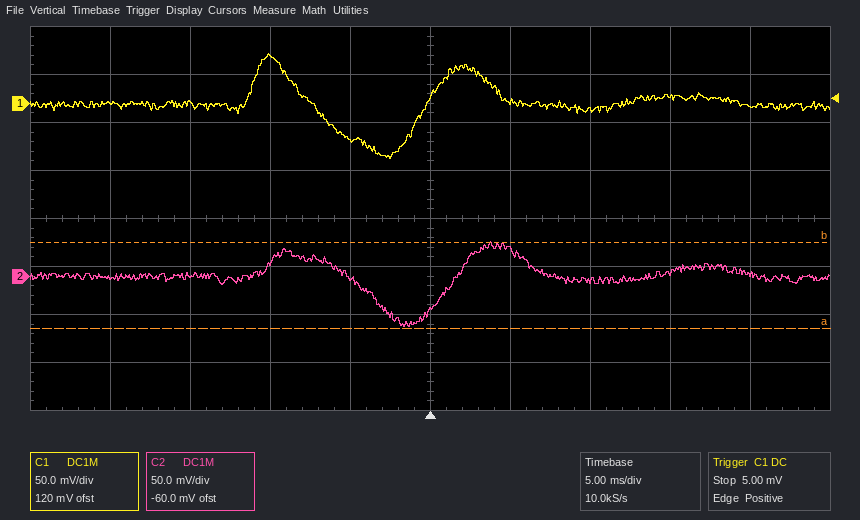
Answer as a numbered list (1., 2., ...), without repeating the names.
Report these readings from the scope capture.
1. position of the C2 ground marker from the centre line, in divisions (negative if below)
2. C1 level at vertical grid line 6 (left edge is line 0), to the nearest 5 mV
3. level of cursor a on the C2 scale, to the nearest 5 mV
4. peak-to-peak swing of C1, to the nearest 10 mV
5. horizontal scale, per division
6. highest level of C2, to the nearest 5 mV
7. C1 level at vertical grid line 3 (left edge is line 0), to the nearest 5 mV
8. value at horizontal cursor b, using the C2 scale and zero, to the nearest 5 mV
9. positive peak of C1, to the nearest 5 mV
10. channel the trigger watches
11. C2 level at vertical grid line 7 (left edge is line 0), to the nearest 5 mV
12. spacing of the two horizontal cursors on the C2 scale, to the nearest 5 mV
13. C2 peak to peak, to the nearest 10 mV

1. -1.2 div
2. 0 mV
3. -55 mV
4. 110 mV
5. 5 ms
6. 35 mV
7. 50 mV
8. 35 mV
9. 50 mV
10. C1
11. -5 mV
12. 90 mV
13. 90 mV
